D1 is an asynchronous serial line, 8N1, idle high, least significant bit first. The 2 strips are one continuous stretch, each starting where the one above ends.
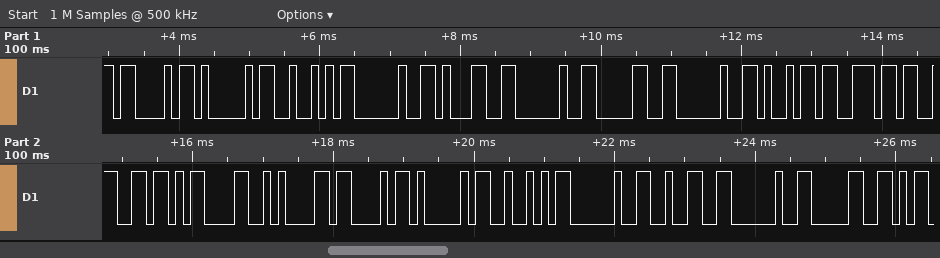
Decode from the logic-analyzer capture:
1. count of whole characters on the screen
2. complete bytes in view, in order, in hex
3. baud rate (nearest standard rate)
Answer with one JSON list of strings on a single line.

["20", "0x43 0x41 0x52 0x20 0x31 0x20 0x30 0x20 0x69 0x6E 0x66 0x0D 0x0A 0x43 0x41 0x52 0x20 0x32 0x20 0x30", "9600 baud"]
